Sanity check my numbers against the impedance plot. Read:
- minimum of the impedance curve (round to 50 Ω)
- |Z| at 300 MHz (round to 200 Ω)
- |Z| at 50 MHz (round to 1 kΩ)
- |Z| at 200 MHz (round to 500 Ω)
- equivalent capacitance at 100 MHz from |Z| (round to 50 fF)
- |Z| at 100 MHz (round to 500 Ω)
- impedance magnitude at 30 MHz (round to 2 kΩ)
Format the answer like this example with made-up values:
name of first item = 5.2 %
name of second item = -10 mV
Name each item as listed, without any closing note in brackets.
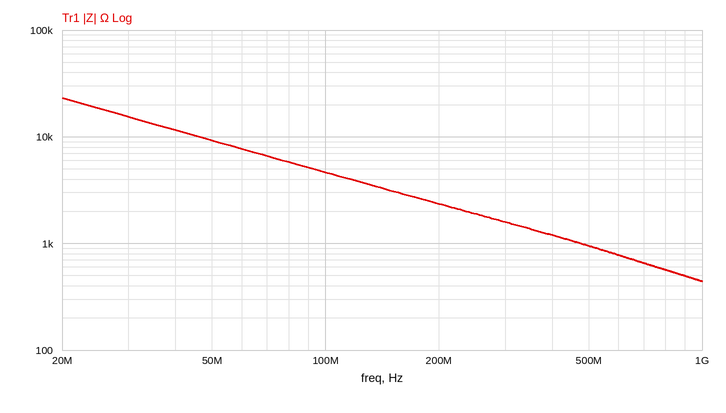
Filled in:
minimum of the impedance curve = 450 Ω
|Z| at 300 MHz = 1.6 kΩ
|Z| at 50 MHz = 9 kΩ
|Z| at 200 MHz = 2.5 kΩ
equivalent capacitance at 100 MHz from |Z| = 350 fF
|Z| at 100 MHz = 4.5 kΩ
impedance magnitude at 30 MHz = 16 kΩ
